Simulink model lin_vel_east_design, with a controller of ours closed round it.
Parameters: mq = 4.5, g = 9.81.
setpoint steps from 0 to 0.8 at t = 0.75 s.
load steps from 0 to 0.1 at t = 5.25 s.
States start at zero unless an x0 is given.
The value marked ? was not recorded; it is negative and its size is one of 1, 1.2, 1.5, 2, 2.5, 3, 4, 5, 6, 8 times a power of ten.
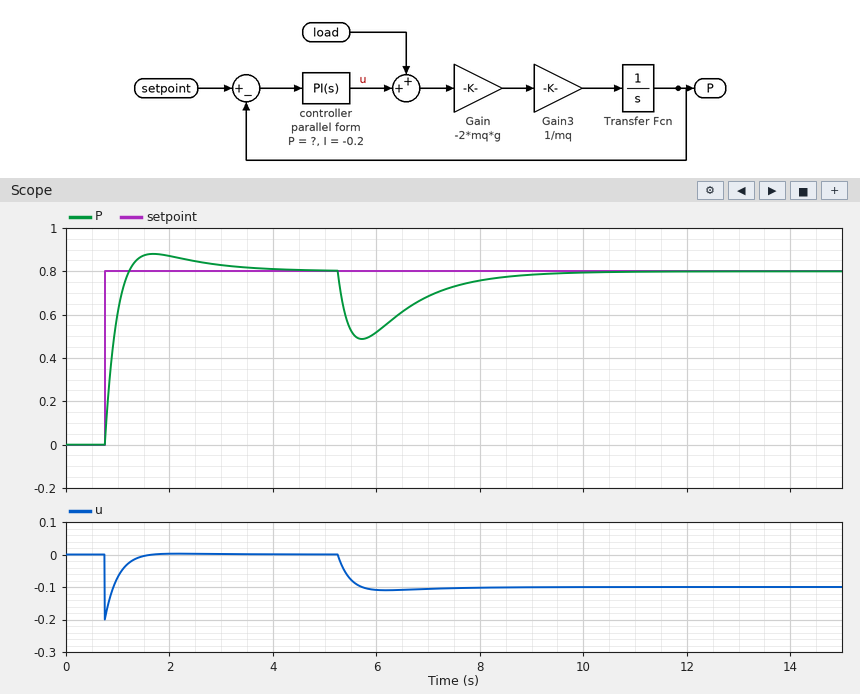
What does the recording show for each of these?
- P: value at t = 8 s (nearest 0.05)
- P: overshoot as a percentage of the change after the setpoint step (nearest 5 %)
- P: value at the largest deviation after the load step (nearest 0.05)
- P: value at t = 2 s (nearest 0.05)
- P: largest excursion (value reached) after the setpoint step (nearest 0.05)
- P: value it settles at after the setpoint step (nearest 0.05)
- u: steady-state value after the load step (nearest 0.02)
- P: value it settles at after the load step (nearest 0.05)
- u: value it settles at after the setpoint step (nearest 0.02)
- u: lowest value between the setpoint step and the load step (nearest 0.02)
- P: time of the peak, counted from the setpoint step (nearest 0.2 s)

0.75
10 %
0.50
0.85
0.90
0.80
-0.10
0.80
0.00
-0.20
1.0 s
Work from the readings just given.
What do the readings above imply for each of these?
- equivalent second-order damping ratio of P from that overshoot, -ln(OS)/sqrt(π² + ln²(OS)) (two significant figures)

0.59
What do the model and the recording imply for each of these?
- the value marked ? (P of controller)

-0.25
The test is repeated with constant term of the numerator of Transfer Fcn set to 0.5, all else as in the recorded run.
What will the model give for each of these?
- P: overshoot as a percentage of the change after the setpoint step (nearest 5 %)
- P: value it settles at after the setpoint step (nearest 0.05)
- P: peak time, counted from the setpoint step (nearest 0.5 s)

15 %
0.80
1.5 s
